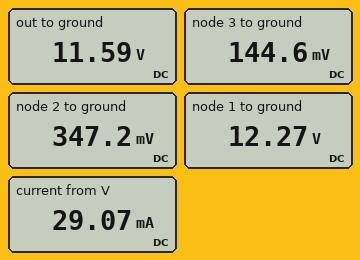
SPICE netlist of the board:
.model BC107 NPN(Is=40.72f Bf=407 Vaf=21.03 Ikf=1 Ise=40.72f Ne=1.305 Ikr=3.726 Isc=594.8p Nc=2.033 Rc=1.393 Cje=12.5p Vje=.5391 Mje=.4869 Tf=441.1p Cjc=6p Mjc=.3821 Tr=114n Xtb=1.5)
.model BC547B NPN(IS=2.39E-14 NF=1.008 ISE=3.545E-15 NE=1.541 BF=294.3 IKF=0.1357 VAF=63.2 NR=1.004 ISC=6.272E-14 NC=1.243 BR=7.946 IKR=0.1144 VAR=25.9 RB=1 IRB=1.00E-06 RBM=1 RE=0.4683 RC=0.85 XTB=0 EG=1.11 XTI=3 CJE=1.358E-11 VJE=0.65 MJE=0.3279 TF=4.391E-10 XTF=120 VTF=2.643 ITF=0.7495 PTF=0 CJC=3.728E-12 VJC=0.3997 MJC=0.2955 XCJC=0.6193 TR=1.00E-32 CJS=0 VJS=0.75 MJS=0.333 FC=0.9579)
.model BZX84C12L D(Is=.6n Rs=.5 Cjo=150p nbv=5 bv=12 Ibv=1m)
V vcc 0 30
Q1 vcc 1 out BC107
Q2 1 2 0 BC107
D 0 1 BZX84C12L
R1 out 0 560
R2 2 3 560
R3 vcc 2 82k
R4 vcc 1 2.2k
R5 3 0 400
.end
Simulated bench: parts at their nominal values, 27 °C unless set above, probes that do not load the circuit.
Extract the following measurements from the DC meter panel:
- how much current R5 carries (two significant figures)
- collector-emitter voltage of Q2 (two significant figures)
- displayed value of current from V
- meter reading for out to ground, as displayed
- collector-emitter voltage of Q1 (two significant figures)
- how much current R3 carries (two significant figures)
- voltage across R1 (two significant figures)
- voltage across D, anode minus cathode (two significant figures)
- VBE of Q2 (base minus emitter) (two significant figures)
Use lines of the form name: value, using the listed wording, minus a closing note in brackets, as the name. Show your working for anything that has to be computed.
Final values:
how much current R5 carries: (144.6 mV) / 400 Ω = 360 µA
collector-emitter voltage of Q2: 12.27 V = 12 V
displayed value of current from V: 29.07 mA
meter reading for out to ground, as displayed: 11.59 V
collector-emitter voltage of Q1: 30 V - 11.59 V = 18 V
how much current R3 carries: (30 V - 347.2 mV) / 82 kΩ = 360 µA
voltage across R1: 11.59 V = 12 V
voltage across D, anode minus cathode: 0 V - 12.27 V = -12 V
VBE of Q2 (base minus emitter): 347.2 mV = 350 mV
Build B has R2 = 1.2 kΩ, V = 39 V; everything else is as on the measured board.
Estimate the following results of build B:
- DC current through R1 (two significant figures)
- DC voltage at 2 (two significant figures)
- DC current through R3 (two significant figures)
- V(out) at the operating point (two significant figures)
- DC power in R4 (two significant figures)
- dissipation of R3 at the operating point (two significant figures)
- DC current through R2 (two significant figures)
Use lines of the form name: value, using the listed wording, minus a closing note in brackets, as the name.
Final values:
DC current through R1: 16 mA
DC voltage at 2: 680 mV
DC current through R3: 470 µA
V(out) at the operating point: 8.9 V
DC power in R4: 390 mW
dissipation of R3 at the operating point: 18 mW
DC current through R2: 420 µA
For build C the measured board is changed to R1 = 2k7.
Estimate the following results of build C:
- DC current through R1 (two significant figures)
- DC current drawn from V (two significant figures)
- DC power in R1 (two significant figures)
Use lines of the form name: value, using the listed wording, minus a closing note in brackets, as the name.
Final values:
DC current through R1: 4.3 mA
DC current drawn from V: 13 mA
DC power in R1: 50 mW
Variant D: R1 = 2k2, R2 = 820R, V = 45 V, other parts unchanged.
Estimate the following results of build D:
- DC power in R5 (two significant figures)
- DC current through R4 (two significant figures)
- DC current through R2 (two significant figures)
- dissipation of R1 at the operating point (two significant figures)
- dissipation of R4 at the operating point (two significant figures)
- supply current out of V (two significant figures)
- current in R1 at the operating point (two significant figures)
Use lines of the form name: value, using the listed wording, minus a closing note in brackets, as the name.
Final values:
DC power in R5: 110 µW
DC current through R4: 15 mA
DC current through R2: 530 µA
dissipation of R1 at the operating point: 62 mW
dissipation of R4 at the operating point: 490 mW
supply current out of V: 21 mA
current in R1 at the operating point: 5.3 mA
